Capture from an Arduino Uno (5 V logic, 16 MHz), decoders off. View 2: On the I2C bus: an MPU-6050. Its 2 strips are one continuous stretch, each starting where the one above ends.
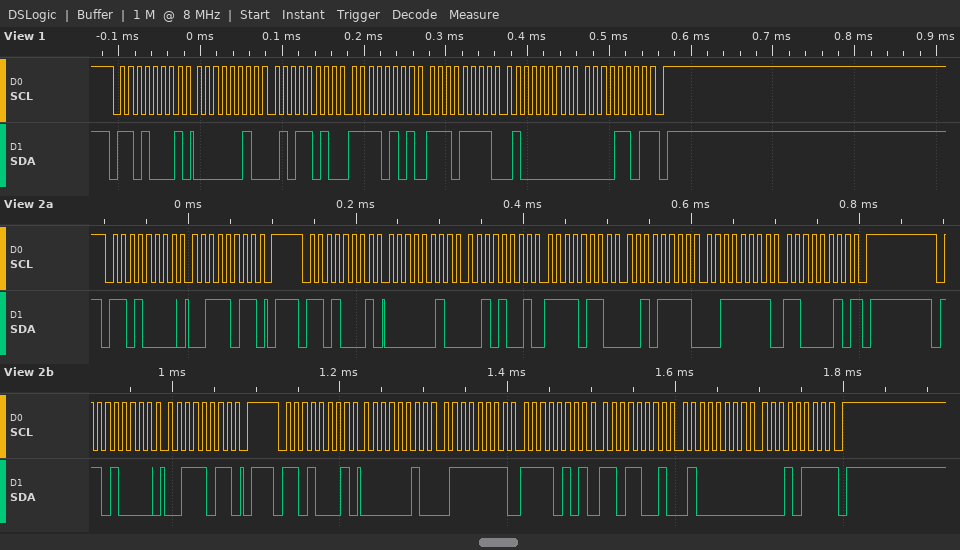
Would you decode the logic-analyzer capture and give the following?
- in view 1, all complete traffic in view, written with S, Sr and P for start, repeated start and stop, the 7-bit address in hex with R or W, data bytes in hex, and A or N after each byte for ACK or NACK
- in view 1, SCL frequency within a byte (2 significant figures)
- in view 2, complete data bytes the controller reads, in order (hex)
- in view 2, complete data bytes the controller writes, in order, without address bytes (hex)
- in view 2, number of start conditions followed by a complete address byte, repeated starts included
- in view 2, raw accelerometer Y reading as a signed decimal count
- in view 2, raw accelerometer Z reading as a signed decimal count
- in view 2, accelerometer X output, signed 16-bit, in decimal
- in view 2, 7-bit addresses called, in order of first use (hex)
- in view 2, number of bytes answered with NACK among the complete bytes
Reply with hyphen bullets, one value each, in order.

- S 68R A 02 A 5A A F5 A EF A 40 A 0D N P
- 100 kHz
- 02 29 F6 2F 3F C2 02 7F F5 D9 40 17
- 3B 3B
- 4
- -2513
- 16322
- 553
- 0x68
- 2
